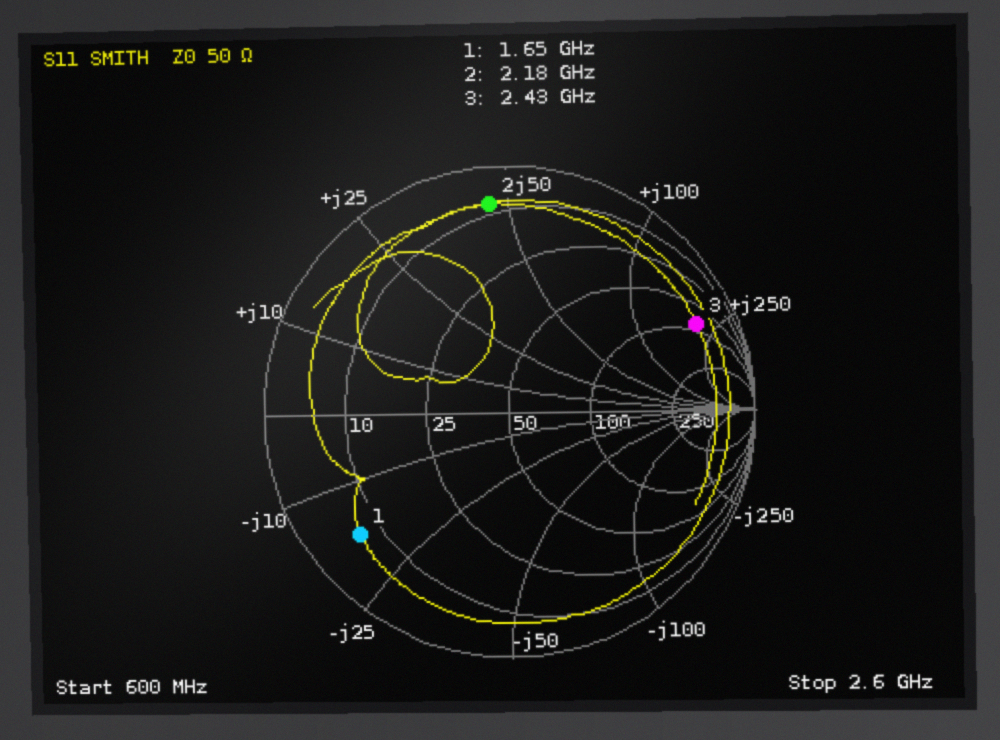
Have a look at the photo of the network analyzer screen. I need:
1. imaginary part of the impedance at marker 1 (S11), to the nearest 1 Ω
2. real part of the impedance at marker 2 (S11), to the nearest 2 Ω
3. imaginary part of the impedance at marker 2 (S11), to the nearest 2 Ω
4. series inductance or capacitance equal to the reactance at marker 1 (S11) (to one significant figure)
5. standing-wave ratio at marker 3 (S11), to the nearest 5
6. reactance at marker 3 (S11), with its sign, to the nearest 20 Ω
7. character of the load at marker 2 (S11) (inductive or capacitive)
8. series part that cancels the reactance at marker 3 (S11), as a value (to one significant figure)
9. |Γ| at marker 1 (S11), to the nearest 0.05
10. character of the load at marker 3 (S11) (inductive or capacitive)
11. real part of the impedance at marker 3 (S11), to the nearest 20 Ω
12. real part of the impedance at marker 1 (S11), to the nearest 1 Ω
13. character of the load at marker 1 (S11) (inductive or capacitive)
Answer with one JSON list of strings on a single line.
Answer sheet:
["-17 Ω", "8 Ω", "+46 Ω", "6 pF", "10", "+200 Ω", "inductive", "300 fF", "0.80", "inductive", "80 Ω", "7 Ω", "capacitive"]
